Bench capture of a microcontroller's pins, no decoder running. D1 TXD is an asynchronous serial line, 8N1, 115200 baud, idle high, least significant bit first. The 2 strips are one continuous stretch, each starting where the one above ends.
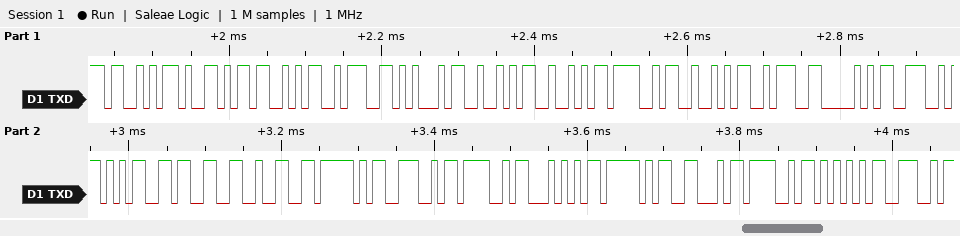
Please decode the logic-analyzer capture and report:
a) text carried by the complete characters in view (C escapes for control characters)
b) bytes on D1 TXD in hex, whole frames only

"SYS:ERROR:PN532_NOT_FOUN"
53 59 53 3A 45 52 52 4F 52 3A 50 4E 35 33 32 5F 4E 4F 54 5F 46 4F 55 4E
